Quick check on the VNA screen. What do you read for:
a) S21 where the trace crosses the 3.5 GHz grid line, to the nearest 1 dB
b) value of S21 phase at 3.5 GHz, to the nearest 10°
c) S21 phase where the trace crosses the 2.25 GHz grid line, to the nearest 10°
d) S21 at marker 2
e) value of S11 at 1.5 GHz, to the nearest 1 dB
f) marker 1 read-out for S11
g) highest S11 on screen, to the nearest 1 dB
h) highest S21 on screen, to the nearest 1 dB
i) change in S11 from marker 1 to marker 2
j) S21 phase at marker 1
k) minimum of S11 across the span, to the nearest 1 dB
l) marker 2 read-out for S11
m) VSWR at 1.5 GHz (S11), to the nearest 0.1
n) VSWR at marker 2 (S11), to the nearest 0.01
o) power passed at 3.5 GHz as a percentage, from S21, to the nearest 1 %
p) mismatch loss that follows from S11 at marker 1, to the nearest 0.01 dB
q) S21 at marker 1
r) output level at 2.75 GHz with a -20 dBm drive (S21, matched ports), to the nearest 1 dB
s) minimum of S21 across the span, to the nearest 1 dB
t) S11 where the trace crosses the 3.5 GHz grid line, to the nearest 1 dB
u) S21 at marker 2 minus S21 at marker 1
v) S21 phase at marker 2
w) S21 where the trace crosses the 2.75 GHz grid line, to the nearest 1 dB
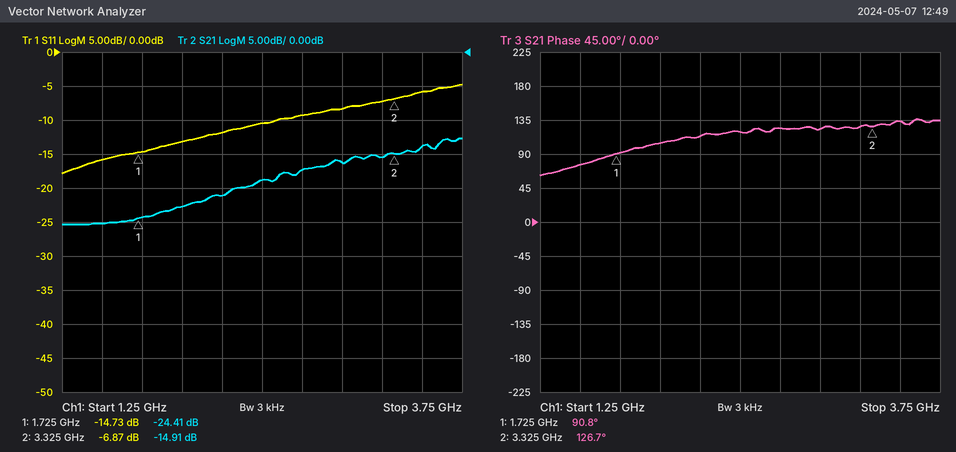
-14 dB
130°
110°
-14.91 dB
-16 dB
-14.73 dB
-5 dB
-13 dB
7.86 dB
90.8°
-18 dB
-6.87 dB
1.4
2.66
4 %
0.15 dB
-24.41 dB
-37 dBm
-25 dB
-6 dB
9.50 dB
126.7°
-17 dB
